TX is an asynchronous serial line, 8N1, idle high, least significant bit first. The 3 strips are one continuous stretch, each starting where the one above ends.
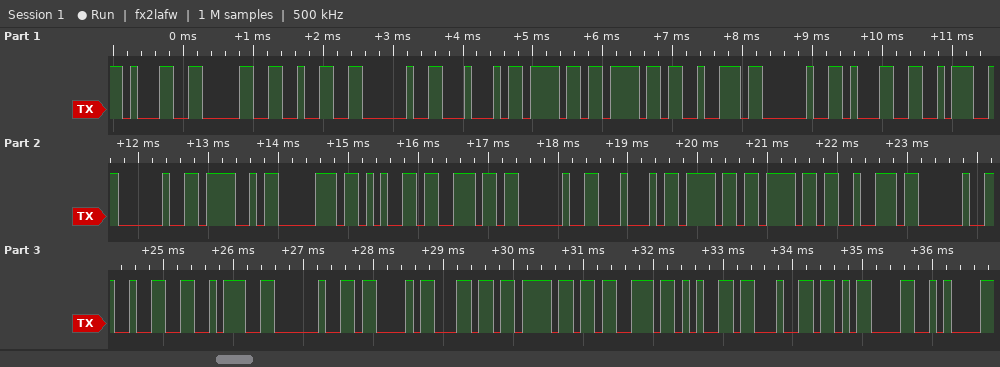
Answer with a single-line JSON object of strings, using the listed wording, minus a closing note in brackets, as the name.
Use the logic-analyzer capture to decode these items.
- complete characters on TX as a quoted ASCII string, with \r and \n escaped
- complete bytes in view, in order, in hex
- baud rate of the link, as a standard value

{"complete characters on TX as a quoted ASCII string, with \\r and \\n escaped": "\"102 Door 1: Open Door 2: Closed\\r\\n\"", "complete bytes in view, in order, in hex": "31 30 32 20 44 6F 6F 72 20 31 3A 20 4F 70 65 6E 20 44 6F 6F 72 20 32 3A 20 43 6C 6F 73 65 64 0D 0A", "baud rate of the link, as a standard value": "9600 baud"}
